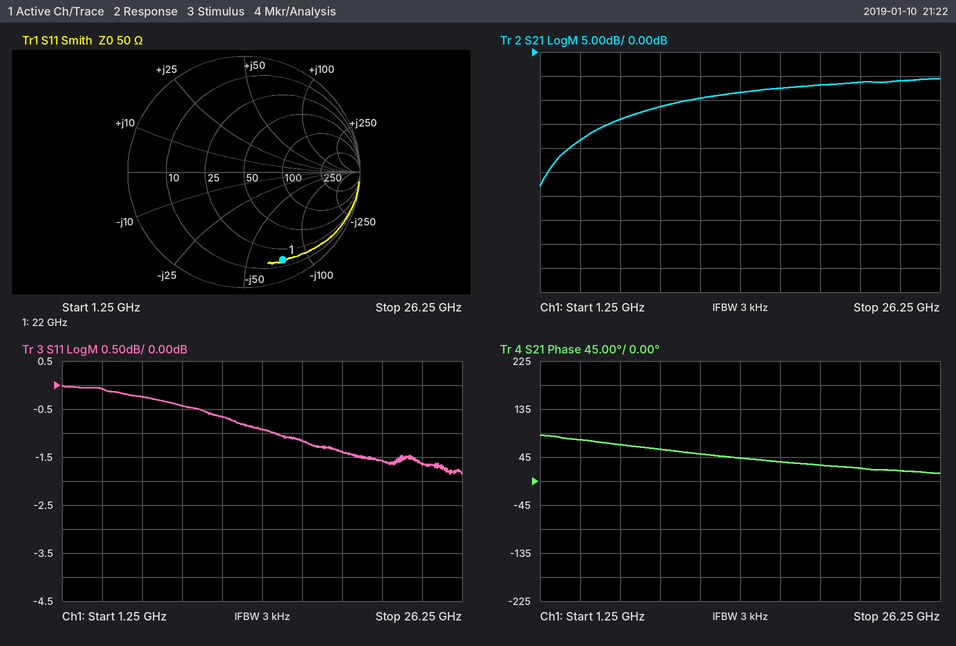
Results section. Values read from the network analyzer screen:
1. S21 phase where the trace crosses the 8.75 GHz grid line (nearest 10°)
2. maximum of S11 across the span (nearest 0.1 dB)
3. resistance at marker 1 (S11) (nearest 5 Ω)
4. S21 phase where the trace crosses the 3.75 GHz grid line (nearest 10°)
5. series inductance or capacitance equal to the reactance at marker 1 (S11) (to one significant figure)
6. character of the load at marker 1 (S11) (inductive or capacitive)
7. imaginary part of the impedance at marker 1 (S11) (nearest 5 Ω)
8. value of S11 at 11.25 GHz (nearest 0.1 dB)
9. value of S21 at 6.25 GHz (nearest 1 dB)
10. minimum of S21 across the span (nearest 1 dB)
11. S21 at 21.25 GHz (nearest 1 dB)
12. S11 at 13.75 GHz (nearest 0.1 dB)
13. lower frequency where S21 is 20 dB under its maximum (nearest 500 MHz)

60°
0.0 dB
15 Ω
80°
100 fF
capacitive
-75 Ω
-0.7 dB
-14 dB
-28 dB
-6 dB
-0.9 dB
1.5 GHz
